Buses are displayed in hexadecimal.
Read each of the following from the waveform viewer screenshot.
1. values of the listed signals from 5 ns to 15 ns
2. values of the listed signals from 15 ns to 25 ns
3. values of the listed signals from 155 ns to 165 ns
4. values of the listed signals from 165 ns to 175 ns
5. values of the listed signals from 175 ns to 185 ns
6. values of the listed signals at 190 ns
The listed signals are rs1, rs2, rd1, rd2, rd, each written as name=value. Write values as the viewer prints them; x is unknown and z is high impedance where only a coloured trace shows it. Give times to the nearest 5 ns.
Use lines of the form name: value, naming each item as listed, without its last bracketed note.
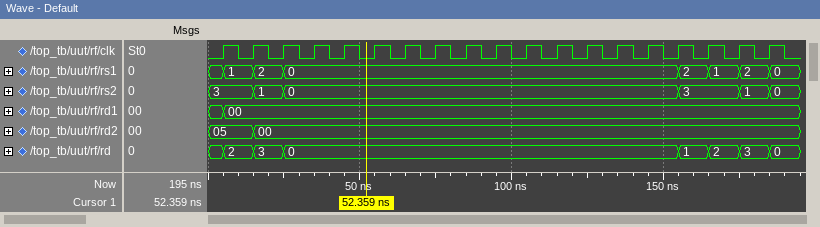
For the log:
values of the listed signals from 5 ns to 15 ns: rs1=1, rs2=3, rd1=00, rd2=05, rd=2
values of the listed signals from 15 ns to 25 ns: rs1=2, rs2=1, rd1=00, rd2=00, rd=3
values of the listed signals from 155 ns to 165 ns: rs1=2, rs2=3, rd1=00, rd2=00, rd=1
values of the listed signals from 165 ns to 175 ns: rs1=1, rs2=3, rd1=00, rd2=00, rd=2
values of the listed signals from 175 ns to 185 ns: rs1=2, rs2=1, rd1=00, rd2=00, rd=3
values of the listed signals at 190 ns: rs1=0, rs2=0, rd1=00, rd2=00, rd=0
